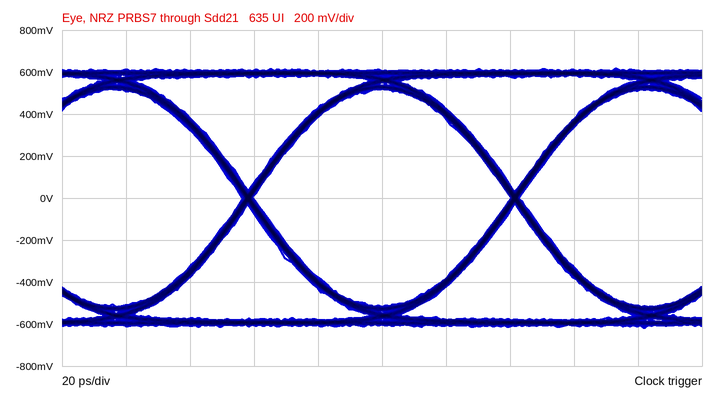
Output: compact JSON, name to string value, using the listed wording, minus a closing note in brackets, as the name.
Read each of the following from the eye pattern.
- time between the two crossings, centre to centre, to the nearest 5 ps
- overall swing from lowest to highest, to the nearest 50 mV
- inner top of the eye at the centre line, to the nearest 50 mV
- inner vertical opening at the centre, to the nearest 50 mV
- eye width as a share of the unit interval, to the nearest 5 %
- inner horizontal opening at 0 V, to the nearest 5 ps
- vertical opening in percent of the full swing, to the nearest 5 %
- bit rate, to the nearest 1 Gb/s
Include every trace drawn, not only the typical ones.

{"time between the two crossings, centre to centre, to the nearest 5 ps": "85 ps", "overall swing from lowest to highest, to the nearest 50 mV": "1.25 V", "inner top of the eye at the centre line, to the nearest 50 mV": "500 mV", "inner vertical opening at the centre, to the nearest 50 mV": "1.05 V", "eye width as a share of the unit interval, to the nearest 5 %": "95 %", "inner horizontal opening at 0 V, to the nearest 5 ps": "80 ps", "vertical opening in percent of the full swing, to the nearest 5 %": "85 %", "bit rate, to the nearest 1 Gb/s": "12 Gb/s"}
